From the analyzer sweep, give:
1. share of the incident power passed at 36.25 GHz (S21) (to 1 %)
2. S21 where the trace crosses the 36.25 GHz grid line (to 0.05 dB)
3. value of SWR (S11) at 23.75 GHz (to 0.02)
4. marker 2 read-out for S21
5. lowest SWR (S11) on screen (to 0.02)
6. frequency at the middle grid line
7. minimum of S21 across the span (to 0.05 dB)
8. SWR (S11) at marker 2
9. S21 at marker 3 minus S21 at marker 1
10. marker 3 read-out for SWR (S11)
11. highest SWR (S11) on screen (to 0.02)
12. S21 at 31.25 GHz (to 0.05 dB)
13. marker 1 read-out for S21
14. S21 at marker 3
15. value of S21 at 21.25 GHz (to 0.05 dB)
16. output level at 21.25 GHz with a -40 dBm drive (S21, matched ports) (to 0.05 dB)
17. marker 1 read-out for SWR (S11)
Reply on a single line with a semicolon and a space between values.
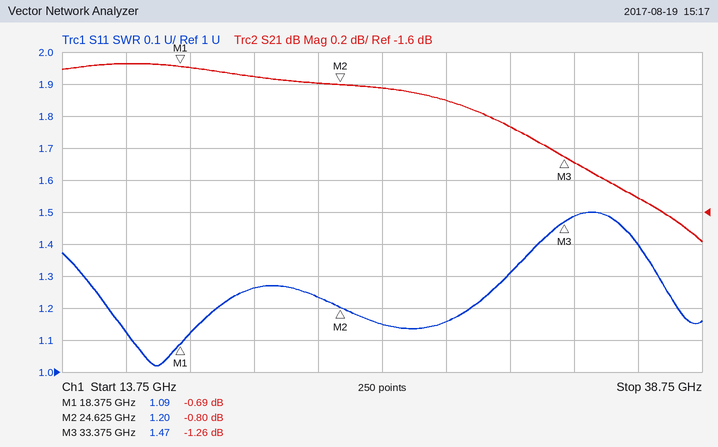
71 %; -1.50 dB; 1.24; -0.80 dB; 1.02; 26.25 GHz; -1.80 dB; 1.20; -0.57 dB; 1.47; 1.50; -1.05 dB; -0.69 dB; -1.26 dB; -0.75 dB; -40.75 dBm; 1.09
